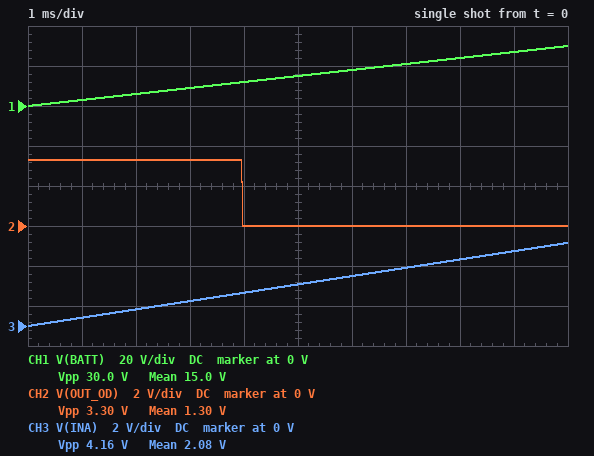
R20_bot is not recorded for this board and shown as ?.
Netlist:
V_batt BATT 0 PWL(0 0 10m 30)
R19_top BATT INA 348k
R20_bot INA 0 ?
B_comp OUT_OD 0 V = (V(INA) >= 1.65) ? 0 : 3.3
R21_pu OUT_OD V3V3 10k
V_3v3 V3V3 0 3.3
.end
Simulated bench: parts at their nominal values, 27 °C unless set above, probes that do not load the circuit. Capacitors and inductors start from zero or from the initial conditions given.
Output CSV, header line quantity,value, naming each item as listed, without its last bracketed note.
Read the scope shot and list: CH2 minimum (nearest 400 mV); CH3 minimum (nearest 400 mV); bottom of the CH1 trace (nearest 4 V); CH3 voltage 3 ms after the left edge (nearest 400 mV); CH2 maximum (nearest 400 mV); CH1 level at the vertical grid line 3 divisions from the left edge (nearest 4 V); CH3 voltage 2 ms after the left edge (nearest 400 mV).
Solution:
quantity,value
CH2 minimum,0 V
CH3 minimum,0 V
bottom of the CH1 trace,0 V
CH3 voltage 3 ms after the left edge,1.2 V
CH2 maximum,3.2 V
CH1 level at the vertical grid line 3 divisions from the left edge,8 V
CH3 voltage 2 ms after the left edge,800 mV
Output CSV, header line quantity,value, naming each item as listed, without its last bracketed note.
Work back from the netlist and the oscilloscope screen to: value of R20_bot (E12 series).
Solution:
quantity,value
value of R20_bot,56 kΩ
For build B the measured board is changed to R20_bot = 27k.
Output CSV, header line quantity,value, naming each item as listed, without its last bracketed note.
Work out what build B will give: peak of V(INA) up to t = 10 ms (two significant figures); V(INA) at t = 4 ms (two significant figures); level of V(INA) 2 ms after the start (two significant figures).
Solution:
quantity,value
peak of V(INA) up to t = 10 ms,2.2 V
V(INA) at t = 4 ms,860 mV
level of V(INA) 2 ms after the start,430 mV
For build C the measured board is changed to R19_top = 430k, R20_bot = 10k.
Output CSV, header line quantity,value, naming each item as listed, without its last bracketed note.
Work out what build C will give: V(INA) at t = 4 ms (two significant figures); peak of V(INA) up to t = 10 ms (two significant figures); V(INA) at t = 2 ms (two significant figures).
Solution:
quantity,value
V(INA) at t = 4 ms,270 mV
peak of V(INA) up to t = 10 ms,680 mV
V(INA) at t = 2 ms,140 mV
